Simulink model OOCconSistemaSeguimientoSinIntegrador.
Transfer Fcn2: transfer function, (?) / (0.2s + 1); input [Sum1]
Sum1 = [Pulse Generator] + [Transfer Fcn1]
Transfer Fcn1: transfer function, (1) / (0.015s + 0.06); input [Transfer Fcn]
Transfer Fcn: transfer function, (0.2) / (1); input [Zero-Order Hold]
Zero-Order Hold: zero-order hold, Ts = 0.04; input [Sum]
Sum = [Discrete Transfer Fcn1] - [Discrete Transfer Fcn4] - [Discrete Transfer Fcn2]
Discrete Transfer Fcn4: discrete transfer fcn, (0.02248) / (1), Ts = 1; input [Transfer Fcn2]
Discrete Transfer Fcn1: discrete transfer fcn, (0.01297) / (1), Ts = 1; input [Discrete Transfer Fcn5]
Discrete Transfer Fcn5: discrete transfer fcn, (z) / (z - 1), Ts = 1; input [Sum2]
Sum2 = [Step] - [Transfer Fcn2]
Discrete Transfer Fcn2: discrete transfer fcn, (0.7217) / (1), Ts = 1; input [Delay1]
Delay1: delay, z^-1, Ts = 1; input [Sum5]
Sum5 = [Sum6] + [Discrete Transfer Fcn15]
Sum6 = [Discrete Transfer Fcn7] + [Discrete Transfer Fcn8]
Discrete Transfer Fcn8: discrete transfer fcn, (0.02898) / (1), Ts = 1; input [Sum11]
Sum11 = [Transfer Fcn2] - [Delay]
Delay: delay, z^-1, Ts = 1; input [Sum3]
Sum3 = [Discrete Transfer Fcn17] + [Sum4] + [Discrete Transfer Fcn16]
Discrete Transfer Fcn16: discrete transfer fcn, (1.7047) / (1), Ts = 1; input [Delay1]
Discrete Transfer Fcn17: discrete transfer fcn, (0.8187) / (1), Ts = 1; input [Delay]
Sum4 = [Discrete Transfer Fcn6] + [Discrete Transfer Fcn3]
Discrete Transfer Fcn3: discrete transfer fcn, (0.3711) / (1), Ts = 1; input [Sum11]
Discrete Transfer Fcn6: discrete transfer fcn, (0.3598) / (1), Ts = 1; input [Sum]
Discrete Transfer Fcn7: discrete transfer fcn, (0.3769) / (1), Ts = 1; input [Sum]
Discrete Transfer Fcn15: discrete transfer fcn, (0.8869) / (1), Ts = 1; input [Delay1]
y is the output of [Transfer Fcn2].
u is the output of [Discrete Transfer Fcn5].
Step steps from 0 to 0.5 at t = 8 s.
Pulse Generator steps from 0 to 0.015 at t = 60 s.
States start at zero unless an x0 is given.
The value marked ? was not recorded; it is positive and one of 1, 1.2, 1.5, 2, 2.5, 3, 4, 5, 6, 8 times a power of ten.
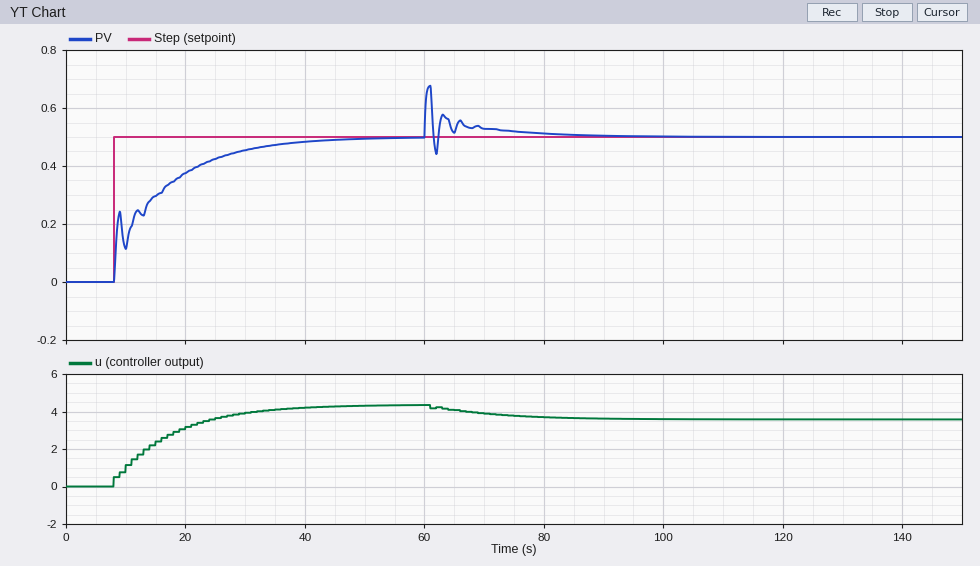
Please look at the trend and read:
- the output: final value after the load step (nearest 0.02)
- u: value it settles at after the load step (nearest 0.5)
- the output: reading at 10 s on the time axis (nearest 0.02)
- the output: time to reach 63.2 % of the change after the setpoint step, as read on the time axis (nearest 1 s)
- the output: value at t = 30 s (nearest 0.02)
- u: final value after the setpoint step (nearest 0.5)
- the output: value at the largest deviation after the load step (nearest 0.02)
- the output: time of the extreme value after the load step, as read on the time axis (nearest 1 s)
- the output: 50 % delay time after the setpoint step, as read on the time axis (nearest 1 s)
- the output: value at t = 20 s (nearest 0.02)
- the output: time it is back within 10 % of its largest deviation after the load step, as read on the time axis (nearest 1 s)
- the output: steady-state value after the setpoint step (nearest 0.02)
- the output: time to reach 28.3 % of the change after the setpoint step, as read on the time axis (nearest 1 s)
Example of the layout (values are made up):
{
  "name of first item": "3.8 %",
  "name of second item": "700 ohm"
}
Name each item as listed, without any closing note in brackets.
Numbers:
{
  "the output: final value after the load step": "0.50",
  "u: value it settles at after the load step": "3.5",
  "the output: reading at 10 s on the time axis": "0.12",
  "the output: time to reach 63.2 % of the change after the setpoint step, as read on the time axis": "16 s",
  "the output: value at t = 30 s": "0.46",
  "u: final value after the setpoint step": "4.5",
  "the output: value at the largest deviation after the load step": "0.68",
  "the output: time of the extreme value after the load step, as read on the time axis": "61 s",
  "the output: 50 % delay time after the setpoint step, as read on the time axis": "13 s",
  "the output: value at t = 20 s": "0.38",
  "the output: time it is back within 10 % of its largest deviation after the load step, as read on the time axis": "76 s",
  "the output: steady-state value after the setpoint step": "0.50",
  "the output: time to reach 28.3 % of the change after the setpoint step, as read on the time axis": "8 s"
}
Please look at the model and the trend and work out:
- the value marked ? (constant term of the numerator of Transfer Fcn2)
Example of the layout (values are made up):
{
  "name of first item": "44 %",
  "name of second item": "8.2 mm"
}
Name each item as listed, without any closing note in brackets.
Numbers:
{
  "the value marked ?": "12"
}
